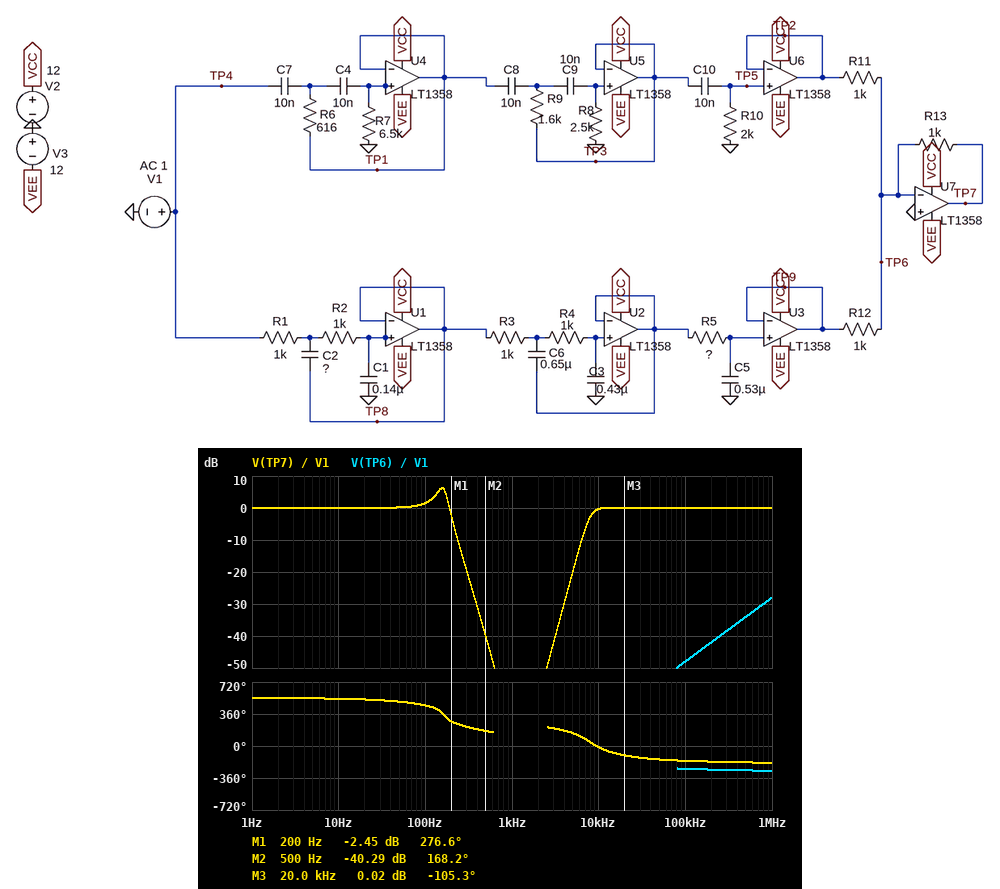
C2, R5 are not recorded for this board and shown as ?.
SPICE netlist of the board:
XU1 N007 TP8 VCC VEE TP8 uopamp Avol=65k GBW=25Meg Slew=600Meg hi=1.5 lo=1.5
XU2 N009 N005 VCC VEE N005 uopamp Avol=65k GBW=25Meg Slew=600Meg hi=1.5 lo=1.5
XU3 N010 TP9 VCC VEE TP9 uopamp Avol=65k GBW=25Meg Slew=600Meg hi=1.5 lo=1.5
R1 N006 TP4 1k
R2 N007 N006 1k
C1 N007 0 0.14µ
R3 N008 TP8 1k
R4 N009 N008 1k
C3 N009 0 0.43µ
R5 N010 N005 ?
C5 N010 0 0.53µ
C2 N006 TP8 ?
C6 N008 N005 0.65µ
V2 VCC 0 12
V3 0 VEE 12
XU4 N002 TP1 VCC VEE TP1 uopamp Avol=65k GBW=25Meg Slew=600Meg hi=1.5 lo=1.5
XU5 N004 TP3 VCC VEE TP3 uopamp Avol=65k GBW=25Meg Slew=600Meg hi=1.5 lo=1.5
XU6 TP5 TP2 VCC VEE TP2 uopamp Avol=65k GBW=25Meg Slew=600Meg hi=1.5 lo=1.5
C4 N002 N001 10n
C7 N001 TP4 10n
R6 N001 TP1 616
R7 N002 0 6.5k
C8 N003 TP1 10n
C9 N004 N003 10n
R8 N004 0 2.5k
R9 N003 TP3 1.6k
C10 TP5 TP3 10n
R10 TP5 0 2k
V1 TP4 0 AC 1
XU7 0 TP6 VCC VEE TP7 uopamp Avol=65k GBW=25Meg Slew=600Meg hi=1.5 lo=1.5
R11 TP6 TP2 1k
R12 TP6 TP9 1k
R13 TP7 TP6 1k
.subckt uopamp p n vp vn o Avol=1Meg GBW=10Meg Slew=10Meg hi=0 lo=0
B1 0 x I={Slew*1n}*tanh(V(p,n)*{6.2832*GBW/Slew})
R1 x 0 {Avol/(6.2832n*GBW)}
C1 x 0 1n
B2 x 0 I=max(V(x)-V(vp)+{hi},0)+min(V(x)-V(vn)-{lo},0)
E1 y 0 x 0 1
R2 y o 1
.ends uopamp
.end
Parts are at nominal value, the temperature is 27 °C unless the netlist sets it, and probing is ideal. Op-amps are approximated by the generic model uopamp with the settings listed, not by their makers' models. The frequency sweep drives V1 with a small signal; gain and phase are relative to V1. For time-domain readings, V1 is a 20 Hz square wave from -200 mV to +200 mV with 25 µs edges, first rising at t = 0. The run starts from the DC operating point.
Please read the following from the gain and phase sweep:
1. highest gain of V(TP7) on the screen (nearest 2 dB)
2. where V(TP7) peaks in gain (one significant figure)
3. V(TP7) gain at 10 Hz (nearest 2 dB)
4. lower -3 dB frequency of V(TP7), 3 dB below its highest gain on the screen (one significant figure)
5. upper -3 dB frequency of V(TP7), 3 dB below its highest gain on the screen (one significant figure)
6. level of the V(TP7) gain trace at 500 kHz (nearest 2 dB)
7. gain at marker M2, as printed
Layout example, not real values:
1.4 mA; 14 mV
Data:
6 dB; 200 Hz; 0 dB; 100 Hz; 200 Hz; 0 dB; -40.29 dB
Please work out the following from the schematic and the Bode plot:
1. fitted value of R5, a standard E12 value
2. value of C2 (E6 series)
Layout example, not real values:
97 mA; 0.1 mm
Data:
2.2 kΩ; 6.8 µF
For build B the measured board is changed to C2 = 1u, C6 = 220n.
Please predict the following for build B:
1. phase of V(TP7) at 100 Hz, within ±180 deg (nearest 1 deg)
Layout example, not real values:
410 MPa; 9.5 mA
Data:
104 deg
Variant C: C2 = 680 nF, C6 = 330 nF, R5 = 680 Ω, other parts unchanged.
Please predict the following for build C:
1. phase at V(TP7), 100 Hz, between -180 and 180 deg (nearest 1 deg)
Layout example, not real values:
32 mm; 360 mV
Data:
127 deg
